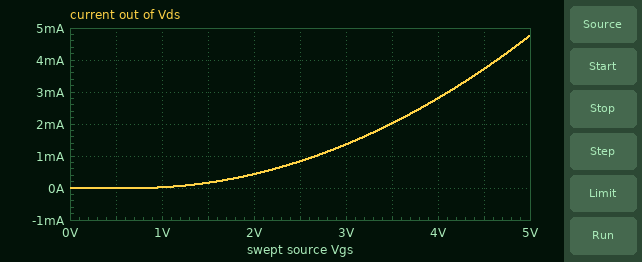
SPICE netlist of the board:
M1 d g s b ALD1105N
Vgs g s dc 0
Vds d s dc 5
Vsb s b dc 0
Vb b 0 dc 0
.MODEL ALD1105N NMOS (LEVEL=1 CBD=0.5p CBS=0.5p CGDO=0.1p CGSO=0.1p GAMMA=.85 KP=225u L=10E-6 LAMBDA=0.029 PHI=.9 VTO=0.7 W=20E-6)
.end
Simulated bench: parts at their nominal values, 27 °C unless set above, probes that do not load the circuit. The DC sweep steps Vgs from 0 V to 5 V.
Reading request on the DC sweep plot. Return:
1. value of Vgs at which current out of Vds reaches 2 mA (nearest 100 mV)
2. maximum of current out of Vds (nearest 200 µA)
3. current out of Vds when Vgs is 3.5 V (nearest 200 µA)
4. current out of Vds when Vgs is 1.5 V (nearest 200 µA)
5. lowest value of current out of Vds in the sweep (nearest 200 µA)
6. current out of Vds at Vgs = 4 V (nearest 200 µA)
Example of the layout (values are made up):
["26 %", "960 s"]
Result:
["3.5 V", "4.8 mA", "2.0 mA", "200 µA", "0 A", "2.8 mA"]
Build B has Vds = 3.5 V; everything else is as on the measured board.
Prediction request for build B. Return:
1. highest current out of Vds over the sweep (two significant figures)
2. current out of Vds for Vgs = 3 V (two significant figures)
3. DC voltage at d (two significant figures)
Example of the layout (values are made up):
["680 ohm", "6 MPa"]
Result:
["4.4 mA", "1.3 mA", "3.5 V"]
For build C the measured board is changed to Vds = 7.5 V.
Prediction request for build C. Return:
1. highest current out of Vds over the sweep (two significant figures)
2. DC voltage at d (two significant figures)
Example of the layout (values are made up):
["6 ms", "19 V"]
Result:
["5.1 mA", "7.5 V"]
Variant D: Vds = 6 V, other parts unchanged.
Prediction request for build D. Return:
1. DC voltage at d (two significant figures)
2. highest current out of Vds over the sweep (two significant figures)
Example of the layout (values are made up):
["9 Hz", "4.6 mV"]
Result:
["6.0 V", "4.9 mA"]
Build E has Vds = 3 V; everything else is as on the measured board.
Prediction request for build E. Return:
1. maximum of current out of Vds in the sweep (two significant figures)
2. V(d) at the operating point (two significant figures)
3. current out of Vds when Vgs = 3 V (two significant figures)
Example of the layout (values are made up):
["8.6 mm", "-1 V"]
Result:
["4.1 mA", "3.0 V", "1.3 mA"]
